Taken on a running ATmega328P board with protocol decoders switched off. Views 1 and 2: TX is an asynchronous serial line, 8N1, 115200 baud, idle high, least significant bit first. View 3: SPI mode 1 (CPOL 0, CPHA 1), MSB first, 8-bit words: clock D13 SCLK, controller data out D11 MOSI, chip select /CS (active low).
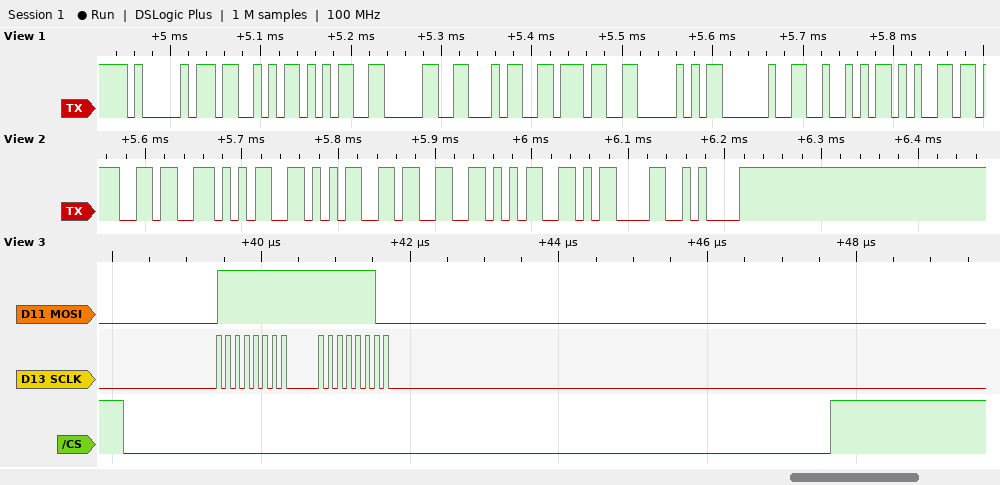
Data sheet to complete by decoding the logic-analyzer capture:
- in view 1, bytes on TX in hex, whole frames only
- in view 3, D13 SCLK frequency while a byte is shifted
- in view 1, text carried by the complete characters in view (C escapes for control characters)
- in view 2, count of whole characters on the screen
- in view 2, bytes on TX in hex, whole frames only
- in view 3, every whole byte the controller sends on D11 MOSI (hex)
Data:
41 53 35 30 34 37 50 20 52 65
8 MHz
"AS5047P Re"
7
0x36 0x35 0x35 0x33 0x35 0x0D 0x0A
FF FC
